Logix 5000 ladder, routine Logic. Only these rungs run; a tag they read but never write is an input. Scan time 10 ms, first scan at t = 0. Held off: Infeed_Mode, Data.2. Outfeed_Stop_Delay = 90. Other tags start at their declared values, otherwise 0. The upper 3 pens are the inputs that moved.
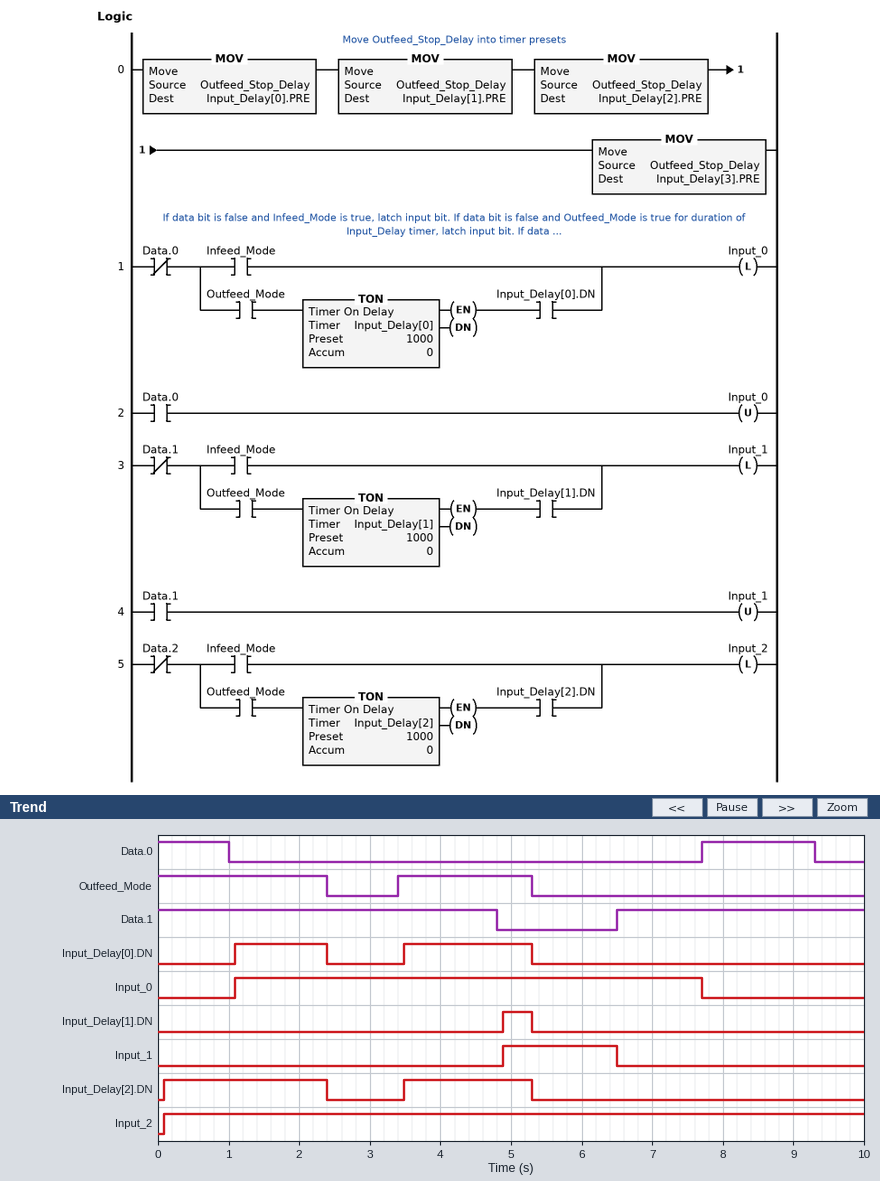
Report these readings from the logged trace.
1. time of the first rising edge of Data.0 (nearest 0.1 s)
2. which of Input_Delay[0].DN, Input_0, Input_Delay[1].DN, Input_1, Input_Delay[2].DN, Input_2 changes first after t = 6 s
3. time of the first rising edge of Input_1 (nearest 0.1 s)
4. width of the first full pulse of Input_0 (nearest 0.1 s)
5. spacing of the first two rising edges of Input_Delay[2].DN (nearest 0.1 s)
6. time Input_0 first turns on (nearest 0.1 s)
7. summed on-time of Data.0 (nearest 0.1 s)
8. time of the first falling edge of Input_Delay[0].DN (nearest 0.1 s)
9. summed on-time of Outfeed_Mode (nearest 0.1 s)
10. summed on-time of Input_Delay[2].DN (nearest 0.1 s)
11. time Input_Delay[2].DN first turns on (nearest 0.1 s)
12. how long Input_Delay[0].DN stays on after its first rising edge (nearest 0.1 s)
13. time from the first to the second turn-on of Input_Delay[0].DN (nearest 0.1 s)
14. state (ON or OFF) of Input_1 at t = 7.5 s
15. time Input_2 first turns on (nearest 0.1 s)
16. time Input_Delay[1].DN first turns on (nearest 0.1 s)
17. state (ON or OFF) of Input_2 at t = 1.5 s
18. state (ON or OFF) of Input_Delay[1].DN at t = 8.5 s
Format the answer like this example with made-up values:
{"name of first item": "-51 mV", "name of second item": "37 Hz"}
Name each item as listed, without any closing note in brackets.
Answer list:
{"time of the first rising edge of Data.0": "7.7 s", "which of Input_Delay[0].DN, Input_0, Input_Delay[1].DN, Input_1, Input_Delay[2].DN, Input_2 changes first after t = 6 s": "Input_1", "time of the first rising edge of Input_1": "4.9 s", "width of the first full pulse of Input_0": "6.6 s", "spacing of the first two rising edges of Input_Delay[2].DN": "3.4 s", "time Input_0 first turns on": "1.1 s", "summed on-time of Data.0": "2.6 s", "time of the first falling edge of Input_Delay[0].DN": "2.4 s", "summed on-time of Outfeed_Mode": "4.3 s", "summed on-time of Input_Delay[2].DN": "4.1 s", "time Input_Delay[2].DN first turns on": "0.1 s", "how long Input_Delay[0].DN stays on after its first rising edge": "1.3 s", "time from the first to the second turn-on of Input_Delay[0].DN": "2.4 s", "state (ON or OFF) of Input_1 at t = 7.5 s": "OFF", "time Input_2 first turns on": "0.1 s", "time Input_Delay[1].DN first turns on": "4.9 s", "state (ON or OFF) of Input_2 at t = 1.5 s": "ON", "state (ON or OFF) of Input_Delay[1].DN at t = 8.5 s": "OFF"}
